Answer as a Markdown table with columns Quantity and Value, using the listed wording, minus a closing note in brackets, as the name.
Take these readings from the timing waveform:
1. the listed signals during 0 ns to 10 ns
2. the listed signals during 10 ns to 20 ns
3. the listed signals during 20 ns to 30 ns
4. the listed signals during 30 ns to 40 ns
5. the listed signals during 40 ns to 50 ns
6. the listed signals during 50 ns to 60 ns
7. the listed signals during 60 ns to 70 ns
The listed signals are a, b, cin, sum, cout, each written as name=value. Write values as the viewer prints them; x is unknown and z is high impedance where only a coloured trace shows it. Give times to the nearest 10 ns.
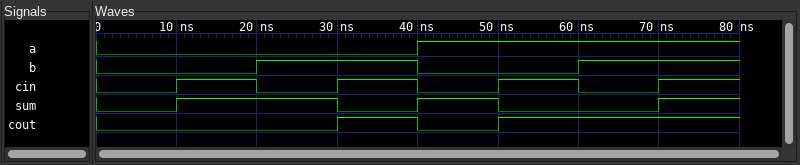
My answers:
| Quantity | Value |
|---|---|
| the listed signals during 0 ns to 10 ns | a=0, b=0, cin=0, sum=0, cout=0 |
| the listed signals during 10 ns to 20 ns | a=0, b=0, cin=1, sum=1, cout=0 |
| the listed signals during 20 ns to 30 ns | a=0, b=1, cin=0, sum=1, cout=0 |
| the listed signals during 30 ns to 40 ns | a=0, b=1, cin=1, sum=0, cout=1 |
| the listed signals during 40 ns to 50 ns | a=1, b=0, cin=0, sum=1, cout=0 |
| the listed signals during 50 ns to 60 ns | a=1, b=0, cin=1, sum=0, cout=1 |
| the listed signals during 60 ns to 70 ns | a=1, b=1, cin=0, sum=0, cout=1 |
